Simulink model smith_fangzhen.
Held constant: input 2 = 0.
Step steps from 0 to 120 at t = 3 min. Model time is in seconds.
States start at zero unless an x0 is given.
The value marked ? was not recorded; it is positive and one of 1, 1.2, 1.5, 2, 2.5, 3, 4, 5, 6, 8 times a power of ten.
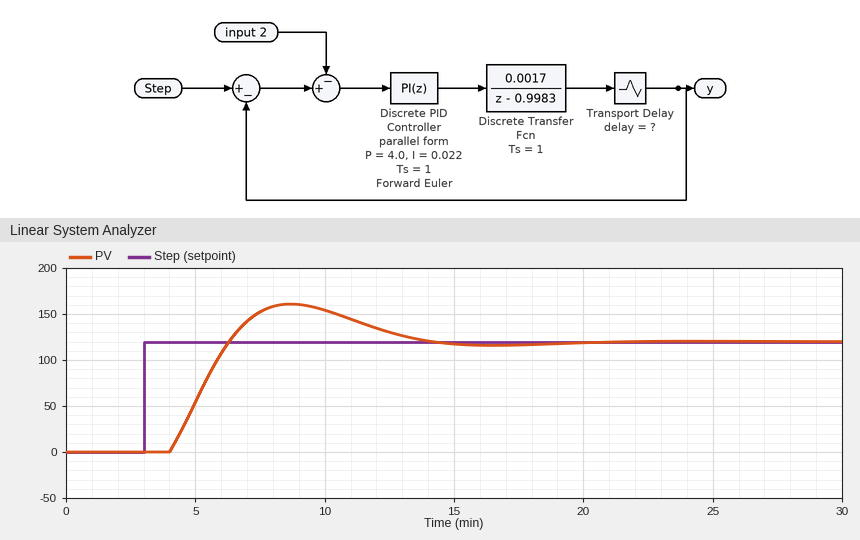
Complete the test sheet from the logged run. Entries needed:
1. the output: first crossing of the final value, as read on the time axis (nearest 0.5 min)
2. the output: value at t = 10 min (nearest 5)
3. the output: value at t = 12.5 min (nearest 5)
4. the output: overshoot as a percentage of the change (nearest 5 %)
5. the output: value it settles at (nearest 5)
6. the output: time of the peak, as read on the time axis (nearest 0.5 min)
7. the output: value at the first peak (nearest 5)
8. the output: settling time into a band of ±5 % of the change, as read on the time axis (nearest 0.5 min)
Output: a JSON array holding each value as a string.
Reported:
["6.5 min", "155", "130", "35 %", "120", "8.5 min", "160", "13.0 min"]
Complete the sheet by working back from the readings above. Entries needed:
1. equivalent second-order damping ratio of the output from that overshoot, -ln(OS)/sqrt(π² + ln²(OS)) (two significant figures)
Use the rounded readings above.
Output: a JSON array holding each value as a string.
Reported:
["0.32"]
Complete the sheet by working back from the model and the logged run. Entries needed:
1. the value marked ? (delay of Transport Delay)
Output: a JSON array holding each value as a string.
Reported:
["60"]
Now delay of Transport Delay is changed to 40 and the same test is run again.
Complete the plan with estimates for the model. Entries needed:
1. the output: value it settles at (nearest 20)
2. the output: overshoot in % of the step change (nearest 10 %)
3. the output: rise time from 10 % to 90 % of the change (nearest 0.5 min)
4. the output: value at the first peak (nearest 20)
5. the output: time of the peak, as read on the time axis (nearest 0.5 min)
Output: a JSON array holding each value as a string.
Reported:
["120", "20 %", "2.0 min", "140", "9.0 min"]
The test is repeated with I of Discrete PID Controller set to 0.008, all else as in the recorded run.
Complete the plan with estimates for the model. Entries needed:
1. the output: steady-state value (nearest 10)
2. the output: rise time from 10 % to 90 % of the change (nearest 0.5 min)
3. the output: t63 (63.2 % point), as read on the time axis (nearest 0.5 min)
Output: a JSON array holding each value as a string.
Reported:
["120", "2.5 min", "5.5 min"]
